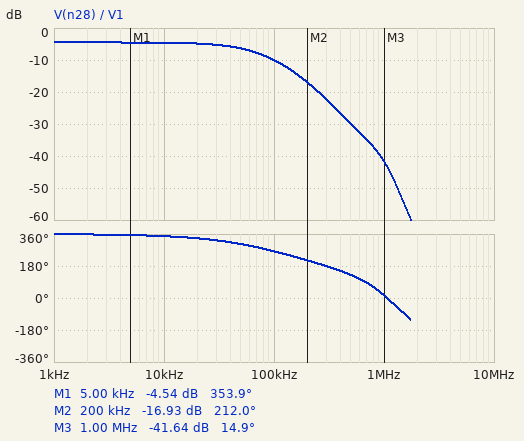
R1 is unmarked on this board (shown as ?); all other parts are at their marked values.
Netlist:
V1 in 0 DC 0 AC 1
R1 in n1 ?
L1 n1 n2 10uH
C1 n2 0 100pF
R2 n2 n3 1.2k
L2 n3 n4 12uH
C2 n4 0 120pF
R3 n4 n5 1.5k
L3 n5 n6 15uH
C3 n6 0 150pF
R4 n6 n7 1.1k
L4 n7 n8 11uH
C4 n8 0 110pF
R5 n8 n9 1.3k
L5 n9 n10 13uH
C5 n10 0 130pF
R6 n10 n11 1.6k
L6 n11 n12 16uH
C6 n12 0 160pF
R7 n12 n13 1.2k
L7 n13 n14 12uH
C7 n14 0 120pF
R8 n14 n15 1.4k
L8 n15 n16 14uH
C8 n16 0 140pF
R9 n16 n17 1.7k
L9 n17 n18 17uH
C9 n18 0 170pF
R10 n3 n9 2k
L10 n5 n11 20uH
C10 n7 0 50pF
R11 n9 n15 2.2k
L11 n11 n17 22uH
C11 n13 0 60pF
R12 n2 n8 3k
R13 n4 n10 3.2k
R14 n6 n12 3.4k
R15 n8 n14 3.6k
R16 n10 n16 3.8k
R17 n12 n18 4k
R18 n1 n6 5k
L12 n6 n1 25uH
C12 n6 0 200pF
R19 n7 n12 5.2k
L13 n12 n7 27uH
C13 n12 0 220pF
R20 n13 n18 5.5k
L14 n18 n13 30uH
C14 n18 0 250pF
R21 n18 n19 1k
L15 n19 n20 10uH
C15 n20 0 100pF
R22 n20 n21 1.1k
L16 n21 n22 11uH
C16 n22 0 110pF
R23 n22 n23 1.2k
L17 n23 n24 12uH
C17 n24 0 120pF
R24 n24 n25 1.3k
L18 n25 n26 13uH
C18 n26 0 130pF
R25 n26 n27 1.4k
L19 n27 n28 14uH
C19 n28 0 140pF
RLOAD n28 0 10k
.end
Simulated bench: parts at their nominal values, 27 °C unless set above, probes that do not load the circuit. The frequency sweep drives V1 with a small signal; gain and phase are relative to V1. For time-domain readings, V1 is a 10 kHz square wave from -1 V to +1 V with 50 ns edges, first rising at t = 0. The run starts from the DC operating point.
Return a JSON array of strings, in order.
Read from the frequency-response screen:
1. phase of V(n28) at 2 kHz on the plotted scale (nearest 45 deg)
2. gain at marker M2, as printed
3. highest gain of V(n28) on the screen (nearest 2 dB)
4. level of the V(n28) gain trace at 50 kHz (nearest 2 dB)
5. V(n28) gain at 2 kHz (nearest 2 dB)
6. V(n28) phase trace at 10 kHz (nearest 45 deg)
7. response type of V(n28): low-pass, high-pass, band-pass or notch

["360 deg", "-16.93 dB", "-4 dB", "-6 dB", "-4 dB", "360 deg", "low-pass"]
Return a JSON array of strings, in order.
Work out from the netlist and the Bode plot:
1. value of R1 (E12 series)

["820 Ω"]
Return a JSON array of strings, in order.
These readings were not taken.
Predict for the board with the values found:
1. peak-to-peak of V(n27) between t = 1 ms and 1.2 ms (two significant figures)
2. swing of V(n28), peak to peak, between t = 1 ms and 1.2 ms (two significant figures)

["1.2 V", "1.2 V"]
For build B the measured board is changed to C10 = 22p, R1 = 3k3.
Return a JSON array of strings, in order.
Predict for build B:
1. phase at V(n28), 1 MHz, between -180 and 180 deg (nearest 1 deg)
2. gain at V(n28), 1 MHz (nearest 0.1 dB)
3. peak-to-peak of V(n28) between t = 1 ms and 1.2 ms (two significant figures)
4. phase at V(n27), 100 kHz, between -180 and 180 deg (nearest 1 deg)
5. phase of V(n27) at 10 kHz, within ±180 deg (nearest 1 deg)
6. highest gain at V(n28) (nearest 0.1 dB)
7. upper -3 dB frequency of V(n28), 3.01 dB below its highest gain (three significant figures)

["18 deg", "-51.6 dB", "1.0 V", "-122 deg", "-27 deg", "-5.7 dB", "23.8 kHz"]
